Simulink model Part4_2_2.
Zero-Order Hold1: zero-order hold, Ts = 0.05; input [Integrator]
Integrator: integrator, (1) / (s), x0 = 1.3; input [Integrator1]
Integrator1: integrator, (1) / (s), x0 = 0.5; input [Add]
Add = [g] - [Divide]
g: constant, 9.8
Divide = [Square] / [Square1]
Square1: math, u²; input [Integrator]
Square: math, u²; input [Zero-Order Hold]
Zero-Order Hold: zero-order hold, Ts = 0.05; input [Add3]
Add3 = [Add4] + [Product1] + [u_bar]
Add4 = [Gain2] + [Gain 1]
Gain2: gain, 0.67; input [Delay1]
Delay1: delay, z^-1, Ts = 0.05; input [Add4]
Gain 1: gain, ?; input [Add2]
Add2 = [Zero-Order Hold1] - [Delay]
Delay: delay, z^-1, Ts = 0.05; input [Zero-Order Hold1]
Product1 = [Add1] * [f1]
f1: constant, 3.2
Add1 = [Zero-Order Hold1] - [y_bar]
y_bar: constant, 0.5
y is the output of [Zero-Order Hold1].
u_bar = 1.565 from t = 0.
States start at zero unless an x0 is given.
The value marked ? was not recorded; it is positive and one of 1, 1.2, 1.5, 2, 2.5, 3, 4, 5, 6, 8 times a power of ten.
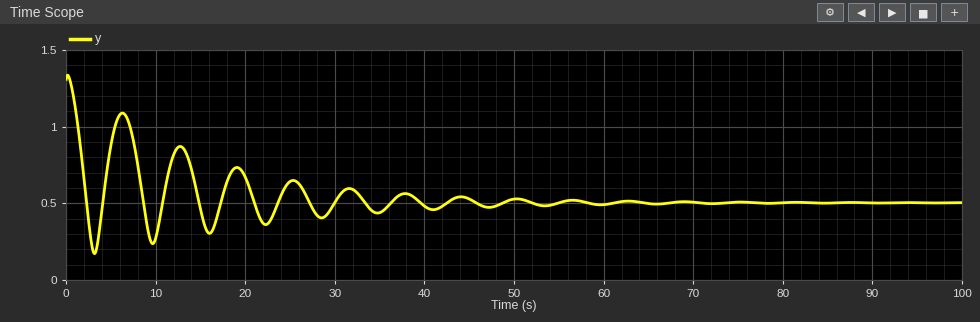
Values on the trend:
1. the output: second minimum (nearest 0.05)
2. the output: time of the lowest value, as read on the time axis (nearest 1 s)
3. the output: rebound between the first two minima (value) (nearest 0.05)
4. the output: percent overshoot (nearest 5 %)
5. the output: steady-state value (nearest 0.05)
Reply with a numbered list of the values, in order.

1. 0.25
2. 3 s
3. 1.10
4. 40 %
5. 0.50
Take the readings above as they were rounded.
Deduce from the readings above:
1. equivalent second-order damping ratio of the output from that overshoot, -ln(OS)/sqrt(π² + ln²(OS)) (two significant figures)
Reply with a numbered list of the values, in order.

1. 0.28
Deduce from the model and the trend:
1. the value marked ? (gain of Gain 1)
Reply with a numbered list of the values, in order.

1. 0.6
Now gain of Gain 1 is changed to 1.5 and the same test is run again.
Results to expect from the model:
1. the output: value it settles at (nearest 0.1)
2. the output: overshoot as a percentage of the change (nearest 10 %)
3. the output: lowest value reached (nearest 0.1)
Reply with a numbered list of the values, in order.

1. 0.5
2. 20 %
3. 0.4
